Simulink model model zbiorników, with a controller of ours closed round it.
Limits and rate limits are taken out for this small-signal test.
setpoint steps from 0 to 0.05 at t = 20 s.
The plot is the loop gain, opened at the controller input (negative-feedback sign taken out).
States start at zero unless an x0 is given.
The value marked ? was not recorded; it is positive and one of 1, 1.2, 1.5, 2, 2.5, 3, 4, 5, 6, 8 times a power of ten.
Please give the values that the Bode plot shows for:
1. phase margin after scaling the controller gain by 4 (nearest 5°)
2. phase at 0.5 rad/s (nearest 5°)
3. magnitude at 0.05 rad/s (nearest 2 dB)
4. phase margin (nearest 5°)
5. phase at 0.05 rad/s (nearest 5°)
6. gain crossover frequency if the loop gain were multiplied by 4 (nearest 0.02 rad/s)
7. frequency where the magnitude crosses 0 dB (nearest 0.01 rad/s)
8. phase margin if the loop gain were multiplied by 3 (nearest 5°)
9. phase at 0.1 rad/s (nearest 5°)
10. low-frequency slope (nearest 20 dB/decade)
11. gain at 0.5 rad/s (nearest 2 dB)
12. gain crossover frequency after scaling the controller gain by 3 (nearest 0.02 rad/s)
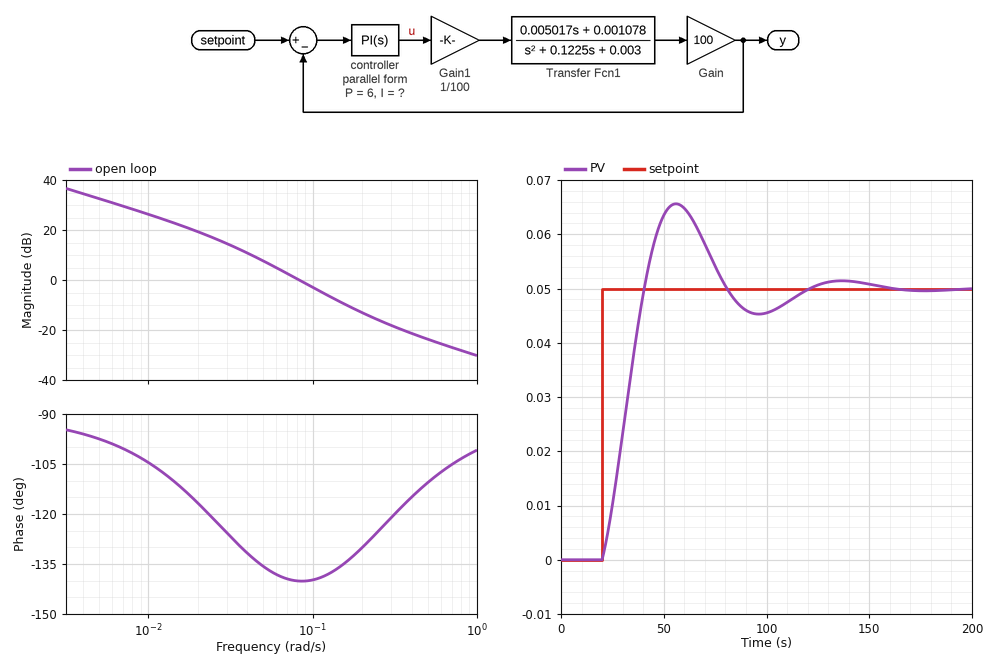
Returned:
50°
-110°
8 dB
40°
-135°
0.18 rad/s
0.08 rad/s
45°
-140°
-20 dB/decade
-24 dB
0.16 rad/s
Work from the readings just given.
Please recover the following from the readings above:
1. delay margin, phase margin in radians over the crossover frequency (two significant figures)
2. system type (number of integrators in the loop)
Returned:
8.7 s
1
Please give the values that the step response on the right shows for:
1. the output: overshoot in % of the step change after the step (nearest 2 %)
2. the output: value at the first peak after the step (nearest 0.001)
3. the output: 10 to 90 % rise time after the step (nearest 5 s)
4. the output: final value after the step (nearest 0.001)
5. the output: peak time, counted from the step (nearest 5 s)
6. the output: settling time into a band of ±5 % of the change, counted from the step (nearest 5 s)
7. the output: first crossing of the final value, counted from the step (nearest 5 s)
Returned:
32 %
0.066
15 s
0.050
35 s
90 s
20 s
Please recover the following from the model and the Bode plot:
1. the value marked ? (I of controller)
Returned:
0.6
